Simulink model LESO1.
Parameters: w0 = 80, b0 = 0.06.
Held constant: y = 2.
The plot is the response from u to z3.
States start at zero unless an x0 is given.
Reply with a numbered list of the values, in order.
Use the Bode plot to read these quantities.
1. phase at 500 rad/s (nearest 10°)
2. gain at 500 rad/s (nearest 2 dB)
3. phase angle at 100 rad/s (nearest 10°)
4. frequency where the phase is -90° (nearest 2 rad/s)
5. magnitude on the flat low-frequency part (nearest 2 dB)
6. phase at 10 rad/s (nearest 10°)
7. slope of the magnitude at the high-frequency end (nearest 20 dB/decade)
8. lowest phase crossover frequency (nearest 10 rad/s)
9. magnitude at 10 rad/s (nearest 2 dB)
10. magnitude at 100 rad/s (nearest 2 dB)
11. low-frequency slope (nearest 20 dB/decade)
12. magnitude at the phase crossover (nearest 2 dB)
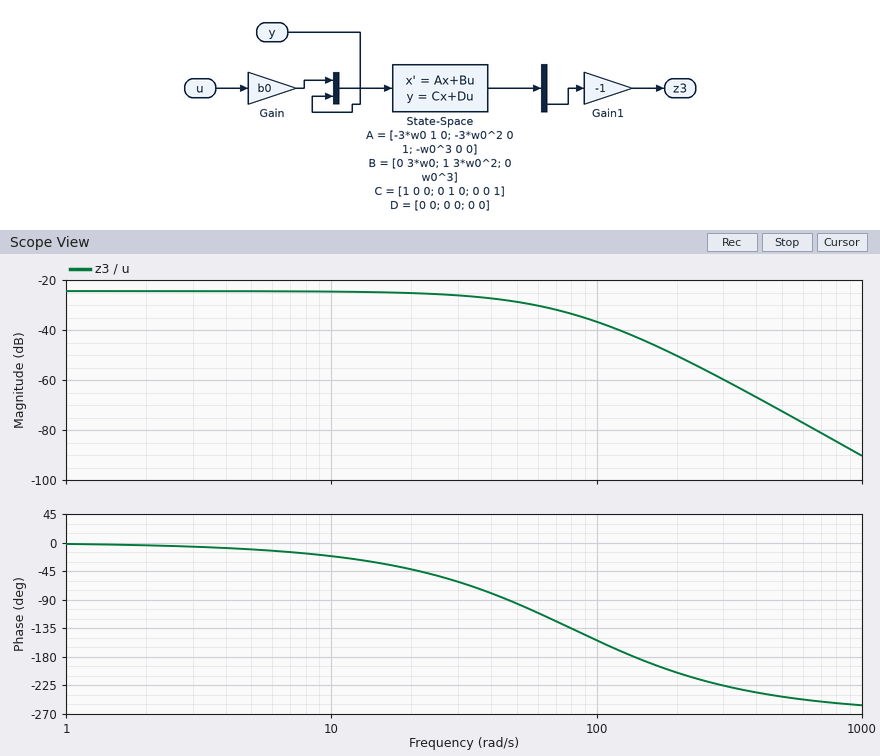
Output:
1. -240°
2. -72 dB
3. -150°
4. 46 rad/s
5. -24 dB
6. -20°
7. -60 dB/decade
8. 140 rad/s
9. -24 dB
10. -36 dB
11. 0 dB/decade
12. -42 dB
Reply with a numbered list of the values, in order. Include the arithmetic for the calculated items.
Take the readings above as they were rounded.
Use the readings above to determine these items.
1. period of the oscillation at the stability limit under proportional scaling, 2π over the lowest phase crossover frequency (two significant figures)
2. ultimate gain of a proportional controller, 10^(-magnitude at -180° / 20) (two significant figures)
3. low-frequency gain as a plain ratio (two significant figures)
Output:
1. 2π / 140 = 0.045 s
2. 10^(42 / 20) = 130
3. 10^(-24 / 20) = 0.063
